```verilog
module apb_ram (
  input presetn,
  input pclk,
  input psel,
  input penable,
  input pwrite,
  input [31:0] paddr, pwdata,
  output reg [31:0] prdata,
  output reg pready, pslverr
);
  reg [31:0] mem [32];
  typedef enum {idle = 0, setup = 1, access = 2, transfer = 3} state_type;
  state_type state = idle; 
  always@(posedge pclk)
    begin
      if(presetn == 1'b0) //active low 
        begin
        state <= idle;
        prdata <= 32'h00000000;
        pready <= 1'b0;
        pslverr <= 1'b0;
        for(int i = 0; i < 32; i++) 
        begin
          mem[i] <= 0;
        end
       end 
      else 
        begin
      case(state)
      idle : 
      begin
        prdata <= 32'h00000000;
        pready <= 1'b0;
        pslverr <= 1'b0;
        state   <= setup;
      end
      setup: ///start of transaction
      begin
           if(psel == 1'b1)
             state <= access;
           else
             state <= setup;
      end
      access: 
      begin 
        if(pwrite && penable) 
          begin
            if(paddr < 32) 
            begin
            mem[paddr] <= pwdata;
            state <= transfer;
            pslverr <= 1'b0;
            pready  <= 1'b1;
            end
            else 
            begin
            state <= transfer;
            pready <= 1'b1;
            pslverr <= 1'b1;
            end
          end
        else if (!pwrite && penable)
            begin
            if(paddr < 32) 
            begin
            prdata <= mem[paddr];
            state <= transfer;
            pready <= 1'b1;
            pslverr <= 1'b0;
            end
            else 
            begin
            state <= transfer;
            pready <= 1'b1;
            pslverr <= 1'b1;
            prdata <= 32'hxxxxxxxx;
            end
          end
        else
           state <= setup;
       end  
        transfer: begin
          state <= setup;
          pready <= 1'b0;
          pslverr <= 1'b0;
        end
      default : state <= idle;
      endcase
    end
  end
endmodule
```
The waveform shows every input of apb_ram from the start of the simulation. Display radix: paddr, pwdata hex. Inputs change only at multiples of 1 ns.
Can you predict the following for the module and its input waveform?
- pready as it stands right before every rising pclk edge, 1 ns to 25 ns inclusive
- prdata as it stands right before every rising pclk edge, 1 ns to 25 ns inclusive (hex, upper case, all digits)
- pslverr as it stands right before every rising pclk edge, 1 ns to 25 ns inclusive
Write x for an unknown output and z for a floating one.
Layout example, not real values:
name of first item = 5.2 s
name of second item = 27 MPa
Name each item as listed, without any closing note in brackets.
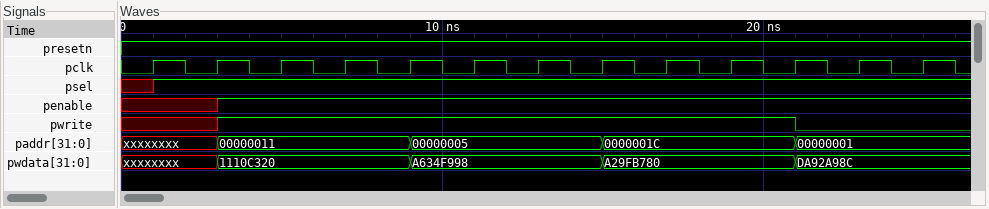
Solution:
pready as it stands right before every rising pclk edge, 1 ns to 25 ns inclusive = x 0 0 1 0 0 1 0 0 1 0 0 1
prdata as it stands right before every rising pclk edge, 1 ns to 25 ns inclusive = x, 00000000, 00000000, 00000000, 00000000, 00000000, 00000000, 00000000, 00000000, 00000000, 00000000, 00000000, x
pslverr as it stands right before every rising pclk edge, 1 ns to 25 ns inclusive = x 0 0 0 0 0 0 0 0 0 0 0 0
